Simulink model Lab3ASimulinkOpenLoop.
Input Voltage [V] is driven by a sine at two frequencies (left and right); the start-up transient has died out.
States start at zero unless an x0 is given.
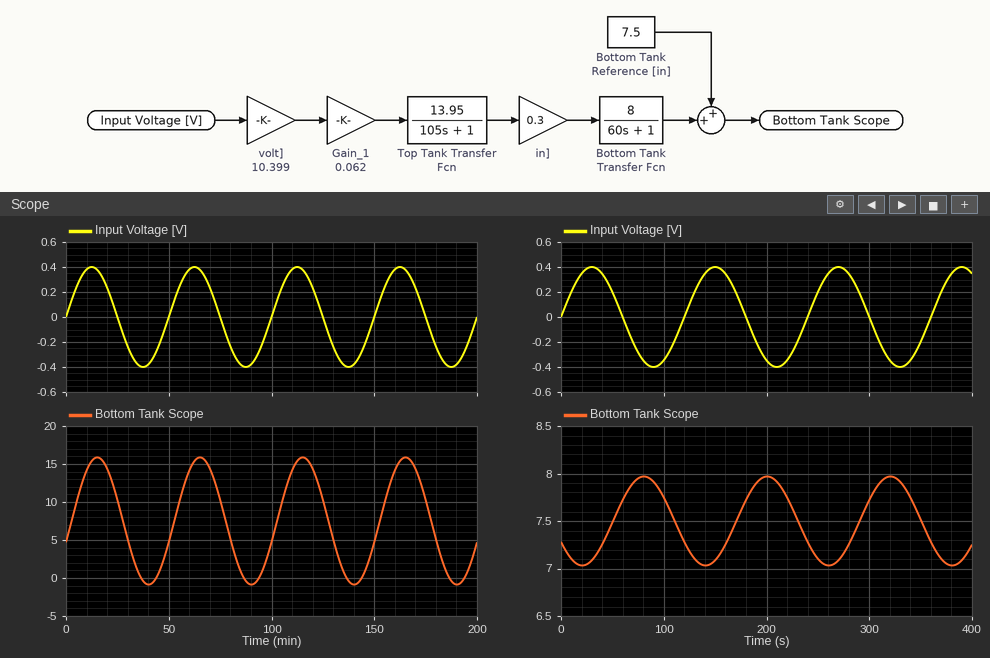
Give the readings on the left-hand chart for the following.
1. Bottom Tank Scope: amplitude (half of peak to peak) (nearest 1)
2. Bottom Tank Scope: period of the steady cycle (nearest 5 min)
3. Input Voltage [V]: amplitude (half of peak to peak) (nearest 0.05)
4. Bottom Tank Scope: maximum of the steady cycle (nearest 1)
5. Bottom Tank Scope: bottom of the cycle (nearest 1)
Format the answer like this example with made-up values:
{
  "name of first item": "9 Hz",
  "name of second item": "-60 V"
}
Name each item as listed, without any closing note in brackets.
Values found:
{
  "Bottom Tank Scope: amplitude (half of peak to peak)": "8",
  "Bottom Tank Scope: period of the steady cycle": "50 min",
  "Input Voltage [V]: amplitude (half of peak to peak)": "0.40",
  "Bottom Tank Scope: maximum of the steady cycle": "16",
  "Bottom Tank Scope: bottom of the cycle": "-1"
}
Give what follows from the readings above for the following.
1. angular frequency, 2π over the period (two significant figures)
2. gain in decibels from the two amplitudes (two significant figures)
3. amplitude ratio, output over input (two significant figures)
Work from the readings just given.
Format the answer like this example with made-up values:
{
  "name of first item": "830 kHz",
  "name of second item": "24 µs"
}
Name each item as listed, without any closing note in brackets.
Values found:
{
  "angular frequency, 2π over the period": "0.13 rad/min",
  "gain in decibels from the two amplitudes": "26 dB",
  "amplitude ratio, output over input": "20"
}
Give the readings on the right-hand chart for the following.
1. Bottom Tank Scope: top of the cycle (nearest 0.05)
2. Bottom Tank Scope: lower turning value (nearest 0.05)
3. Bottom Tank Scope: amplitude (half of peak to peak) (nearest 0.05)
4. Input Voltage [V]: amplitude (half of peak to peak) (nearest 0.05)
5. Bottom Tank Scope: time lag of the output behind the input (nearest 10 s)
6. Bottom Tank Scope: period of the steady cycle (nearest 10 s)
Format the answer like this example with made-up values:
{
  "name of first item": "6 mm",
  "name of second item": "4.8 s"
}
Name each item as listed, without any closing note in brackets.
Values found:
{
  "Bottom Tank Scope: top of the cycle": "7.95",
  "Bottom Tank Scope: lower turning value": "7.05",
  "Bottom Tank Scope: amplitude (half of peak to peak)": "0.45",
  "Input Voltage [V]: amplitude (half of peak to peak)": "0.40",
  "Bottom Tank Scope: time lag of the output behind the input": "50 s",
  "Bottom Tank Scope: period of the steady cycle": "120 s"
}
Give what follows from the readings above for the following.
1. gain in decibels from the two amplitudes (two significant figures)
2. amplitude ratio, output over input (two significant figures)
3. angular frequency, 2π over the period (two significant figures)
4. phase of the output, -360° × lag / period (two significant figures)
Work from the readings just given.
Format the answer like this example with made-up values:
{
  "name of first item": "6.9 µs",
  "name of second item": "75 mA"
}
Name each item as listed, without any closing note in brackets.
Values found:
{
  "gain in decibels from the two amplitudes": "1.0 dB",
  "amplitude ratio, output over input": "1.1",
  "angular frequency, 2π over the period": "0.052 rad/s",
  "phase of the output, -360° × lag / period": "-150°"
}
